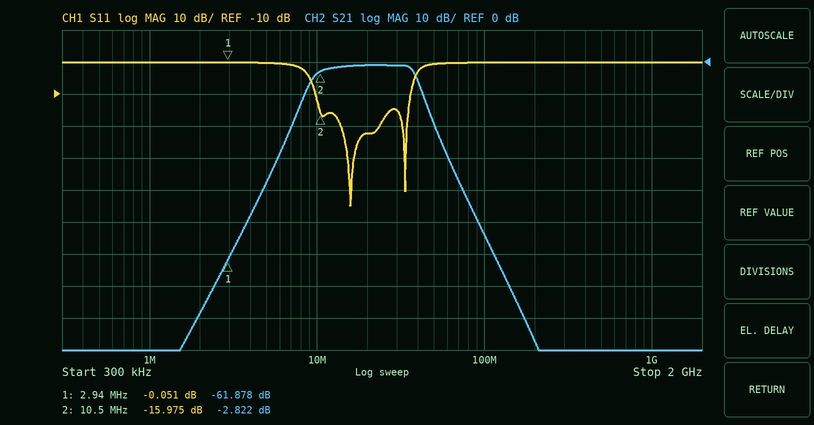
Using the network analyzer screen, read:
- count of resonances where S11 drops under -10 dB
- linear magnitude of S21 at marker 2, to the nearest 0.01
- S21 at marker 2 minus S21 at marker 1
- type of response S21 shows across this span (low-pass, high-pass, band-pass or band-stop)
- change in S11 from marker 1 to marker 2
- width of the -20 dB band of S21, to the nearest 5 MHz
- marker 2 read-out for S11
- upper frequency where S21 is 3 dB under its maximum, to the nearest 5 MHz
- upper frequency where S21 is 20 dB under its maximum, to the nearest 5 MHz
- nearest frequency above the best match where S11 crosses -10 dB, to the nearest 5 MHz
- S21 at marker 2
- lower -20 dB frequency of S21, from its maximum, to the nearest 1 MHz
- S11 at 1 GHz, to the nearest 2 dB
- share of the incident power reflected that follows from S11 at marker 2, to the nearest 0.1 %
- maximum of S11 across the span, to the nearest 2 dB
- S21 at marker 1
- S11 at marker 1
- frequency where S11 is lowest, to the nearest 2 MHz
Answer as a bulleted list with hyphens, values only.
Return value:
- 2
- 0.72
- 59.056 dB
- band-pass
- -15.924 dB
- 45 MHz
- -15.975 dB
- 40 MHz
- 50 MHz
- 35 MHz
- -2.822 dB
- 7 MHz
- 0 dB
- 2.5 %
- 0 dB
- -61.878 dB
- -0.051 dB
- 16 MHz
